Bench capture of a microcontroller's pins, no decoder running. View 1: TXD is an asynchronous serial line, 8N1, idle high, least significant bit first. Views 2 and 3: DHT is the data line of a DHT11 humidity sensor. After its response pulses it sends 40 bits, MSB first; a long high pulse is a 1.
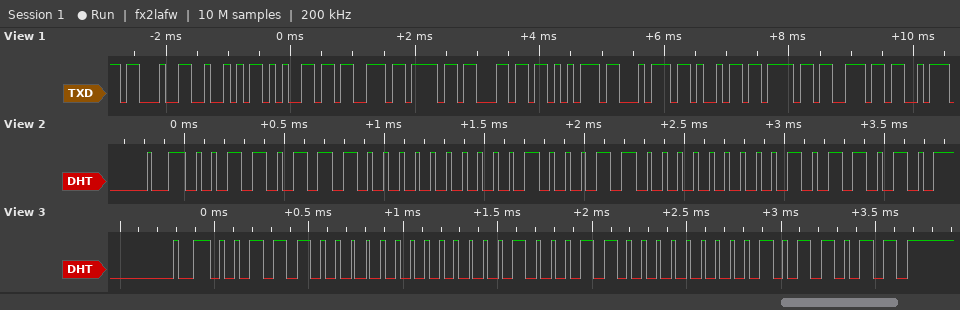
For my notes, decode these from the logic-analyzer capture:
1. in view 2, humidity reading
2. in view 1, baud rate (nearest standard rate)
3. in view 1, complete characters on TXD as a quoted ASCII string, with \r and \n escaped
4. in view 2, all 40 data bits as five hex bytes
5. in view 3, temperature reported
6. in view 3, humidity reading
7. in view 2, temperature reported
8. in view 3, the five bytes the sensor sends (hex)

55 %
9600 baud
"#Resolution"
37 00 23 00 5A
35.0 °C
56 %
35.0 °C
38 00 23 00 5B
